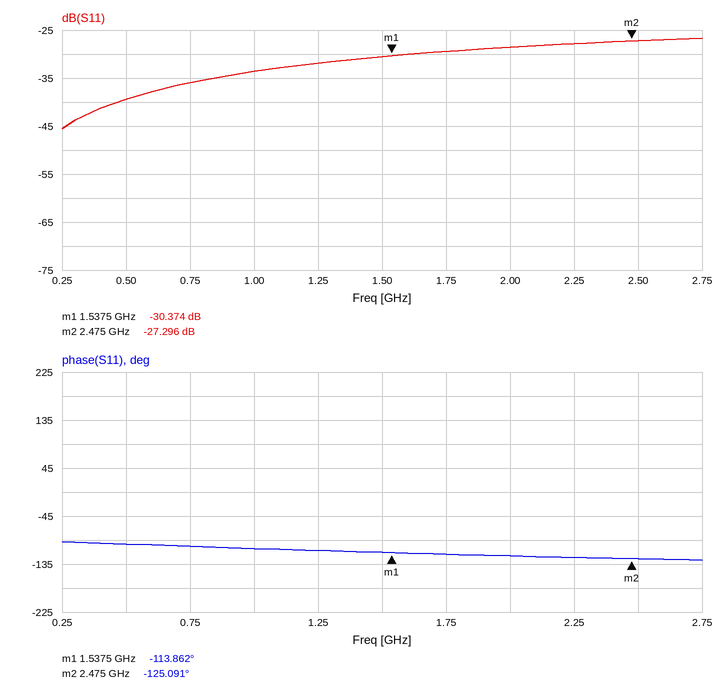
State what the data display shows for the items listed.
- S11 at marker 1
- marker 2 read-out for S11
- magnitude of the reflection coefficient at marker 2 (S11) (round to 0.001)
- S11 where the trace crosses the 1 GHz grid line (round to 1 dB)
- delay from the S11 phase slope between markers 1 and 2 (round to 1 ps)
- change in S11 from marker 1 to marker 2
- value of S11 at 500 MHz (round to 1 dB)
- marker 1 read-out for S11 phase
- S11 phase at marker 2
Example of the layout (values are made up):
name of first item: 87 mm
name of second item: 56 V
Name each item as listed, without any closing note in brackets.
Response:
S11 at marker 1: -30.374 dB
marker 2 read-out for S11: -27.296 dB
magnitude of the reflection coefficient at marker 2 (S11): 0.043
S11 where the trace crosses the 1 GHz grid line: -34 dB
delay from the S11 phase slope between markers 1 and 2: 33 ps
change in S11 from marker 1 to marker 2: 3.078 dB
value of S11 at 500 MHz: -39 dB
marker 1 read-out for S11 phase: -113.862°
S11 phase at marker 2: -125.091°
